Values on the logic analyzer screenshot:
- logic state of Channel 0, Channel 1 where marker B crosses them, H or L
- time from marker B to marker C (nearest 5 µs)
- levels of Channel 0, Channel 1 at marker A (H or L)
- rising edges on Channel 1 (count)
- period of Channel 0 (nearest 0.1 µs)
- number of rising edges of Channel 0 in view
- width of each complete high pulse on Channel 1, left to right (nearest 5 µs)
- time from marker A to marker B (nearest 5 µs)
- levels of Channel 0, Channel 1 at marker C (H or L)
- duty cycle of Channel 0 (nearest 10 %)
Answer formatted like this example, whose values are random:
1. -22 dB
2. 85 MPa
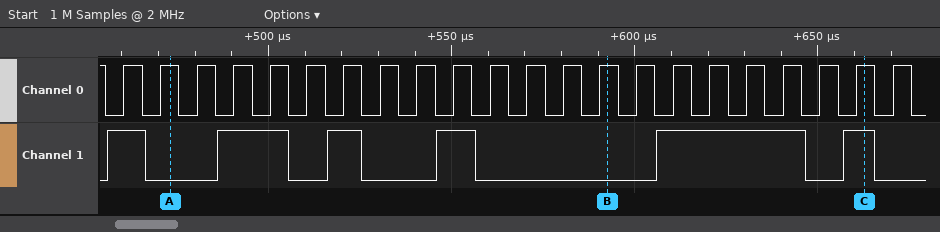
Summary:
1. Channel 0=H, Channel 1=L
2. 70 µs
3. Channel 0=H, Channel 1=L
4. 6
5. 10 µs
6. 22
7. 10 µs, 20 µs, 10 µs, 10 µs, 40 µs, 10 µs
8. 120 µs
9. Channel 0=H, Channel 1=H
10. 50 %
